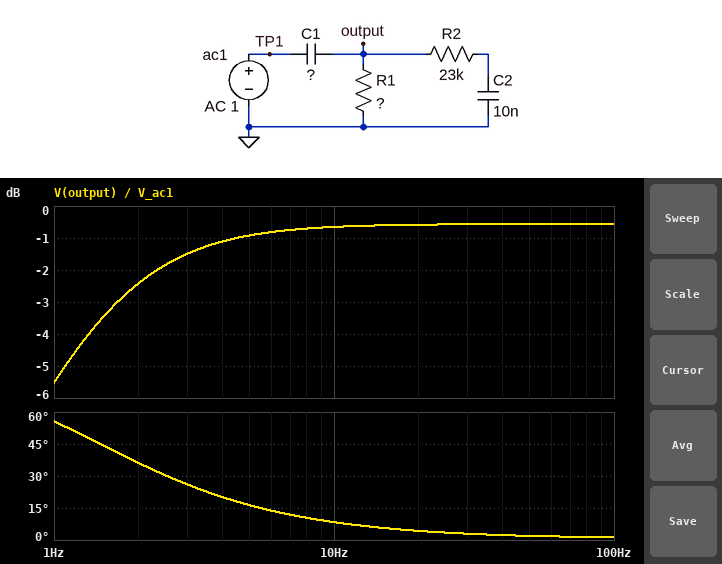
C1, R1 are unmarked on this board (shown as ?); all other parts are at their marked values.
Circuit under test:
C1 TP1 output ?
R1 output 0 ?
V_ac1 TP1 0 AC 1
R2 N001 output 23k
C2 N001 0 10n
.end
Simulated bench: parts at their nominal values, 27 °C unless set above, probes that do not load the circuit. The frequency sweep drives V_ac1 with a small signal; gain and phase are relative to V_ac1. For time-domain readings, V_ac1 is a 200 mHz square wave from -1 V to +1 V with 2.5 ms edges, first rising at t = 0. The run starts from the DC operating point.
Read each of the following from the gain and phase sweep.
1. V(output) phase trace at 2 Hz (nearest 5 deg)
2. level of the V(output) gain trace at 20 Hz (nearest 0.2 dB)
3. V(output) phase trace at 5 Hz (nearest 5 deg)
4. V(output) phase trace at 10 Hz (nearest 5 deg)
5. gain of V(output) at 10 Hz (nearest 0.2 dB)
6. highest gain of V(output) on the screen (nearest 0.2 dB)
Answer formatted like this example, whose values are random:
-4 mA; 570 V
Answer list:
35 deg; -0.6 dB; 15 deg; 10 deg; -0.6 dB; -0.6 dB
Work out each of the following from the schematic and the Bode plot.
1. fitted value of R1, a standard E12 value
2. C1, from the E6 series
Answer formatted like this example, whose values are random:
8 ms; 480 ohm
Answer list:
680 kΩ; 150 nF
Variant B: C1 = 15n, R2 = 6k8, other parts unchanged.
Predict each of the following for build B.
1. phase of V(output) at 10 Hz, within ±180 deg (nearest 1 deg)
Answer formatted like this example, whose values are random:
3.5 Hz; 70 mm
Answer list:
43 deg
